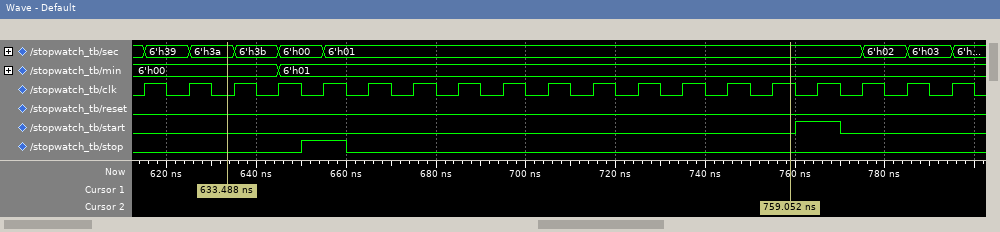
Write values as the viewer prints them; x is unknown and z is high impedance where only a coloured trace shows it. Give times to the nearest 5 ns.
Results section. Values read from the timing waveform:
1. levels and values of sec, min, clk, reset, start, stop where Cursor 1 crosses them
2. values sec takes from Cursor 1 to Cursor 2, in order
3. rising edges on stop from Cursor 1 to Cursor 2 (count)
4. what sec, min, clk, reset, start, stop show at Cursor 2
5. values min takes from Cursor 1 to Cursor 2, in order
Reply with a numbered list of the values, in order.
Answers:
1. sec=6'h3a, min=6'h00, clk=0, reset=0, start=0, stop=0
2. 6'h3a, 6'h3b, 6'h00, 6'h01
3. 1
4. sec=6'h01, min=6'h01, clk=1, reset=0, start=0, stop=0
5. 6'h00, 6'h01
